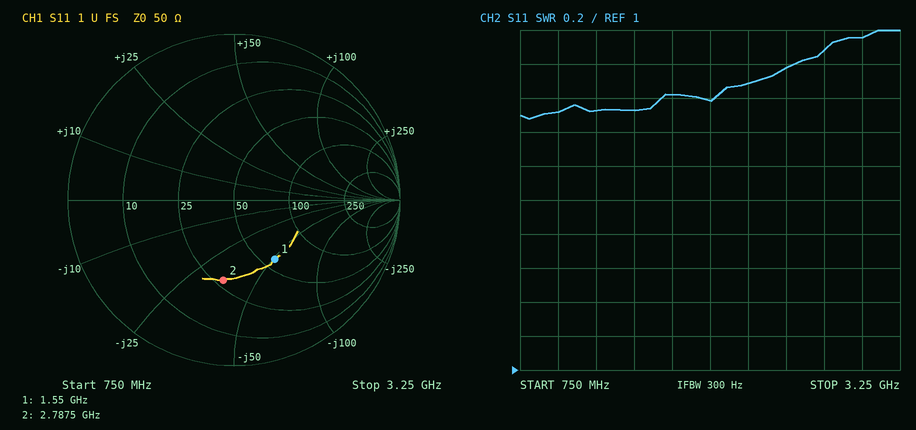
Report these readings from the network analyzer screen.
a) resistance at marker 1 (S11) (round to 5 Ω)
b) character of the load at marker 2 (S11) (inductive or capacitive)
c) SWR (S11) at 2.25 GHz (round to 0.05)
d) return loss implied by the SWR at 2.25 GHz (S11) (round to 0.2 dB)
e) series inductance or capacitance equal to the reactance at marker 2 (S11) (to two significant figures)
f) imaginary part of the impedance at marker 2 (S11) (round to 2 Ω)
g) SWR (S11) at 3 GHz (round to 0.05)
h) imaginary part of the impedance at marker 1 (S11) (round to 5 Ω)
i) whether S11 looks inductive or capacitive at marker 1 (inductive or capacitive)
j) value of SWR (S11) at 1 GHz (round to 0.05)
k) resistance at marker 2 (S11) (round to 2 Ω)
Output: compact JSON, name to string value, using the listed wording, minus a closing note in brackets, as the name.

{"resistance at marker 1 (S11)": "60 Ω", "character of the load at marker 2 (S11)": "capacitive", "SWR (S11) at 2.25 GHz": "2.70", "return loss implied by the SWR at 2.25 GHz (S11)": "6.8 dB", "series inductance or capacitance equal to the reactance at marker 2 (S11)": "1.6 pF", "imaginary part of the impedance at marker 2 (S11)": "-36 Ω", "SWR (S11) at 3 GHz": "2.95", "imaginary part of the impedance at marker 1 (S11)": "-50 Ω", "whether S11 looks inductive or capacitive at marker 1": "capacitive", "value of SWR (S11) at 1 GHz": "2.50", "resistance at marker 2 (S11)": "28 Ω"}
